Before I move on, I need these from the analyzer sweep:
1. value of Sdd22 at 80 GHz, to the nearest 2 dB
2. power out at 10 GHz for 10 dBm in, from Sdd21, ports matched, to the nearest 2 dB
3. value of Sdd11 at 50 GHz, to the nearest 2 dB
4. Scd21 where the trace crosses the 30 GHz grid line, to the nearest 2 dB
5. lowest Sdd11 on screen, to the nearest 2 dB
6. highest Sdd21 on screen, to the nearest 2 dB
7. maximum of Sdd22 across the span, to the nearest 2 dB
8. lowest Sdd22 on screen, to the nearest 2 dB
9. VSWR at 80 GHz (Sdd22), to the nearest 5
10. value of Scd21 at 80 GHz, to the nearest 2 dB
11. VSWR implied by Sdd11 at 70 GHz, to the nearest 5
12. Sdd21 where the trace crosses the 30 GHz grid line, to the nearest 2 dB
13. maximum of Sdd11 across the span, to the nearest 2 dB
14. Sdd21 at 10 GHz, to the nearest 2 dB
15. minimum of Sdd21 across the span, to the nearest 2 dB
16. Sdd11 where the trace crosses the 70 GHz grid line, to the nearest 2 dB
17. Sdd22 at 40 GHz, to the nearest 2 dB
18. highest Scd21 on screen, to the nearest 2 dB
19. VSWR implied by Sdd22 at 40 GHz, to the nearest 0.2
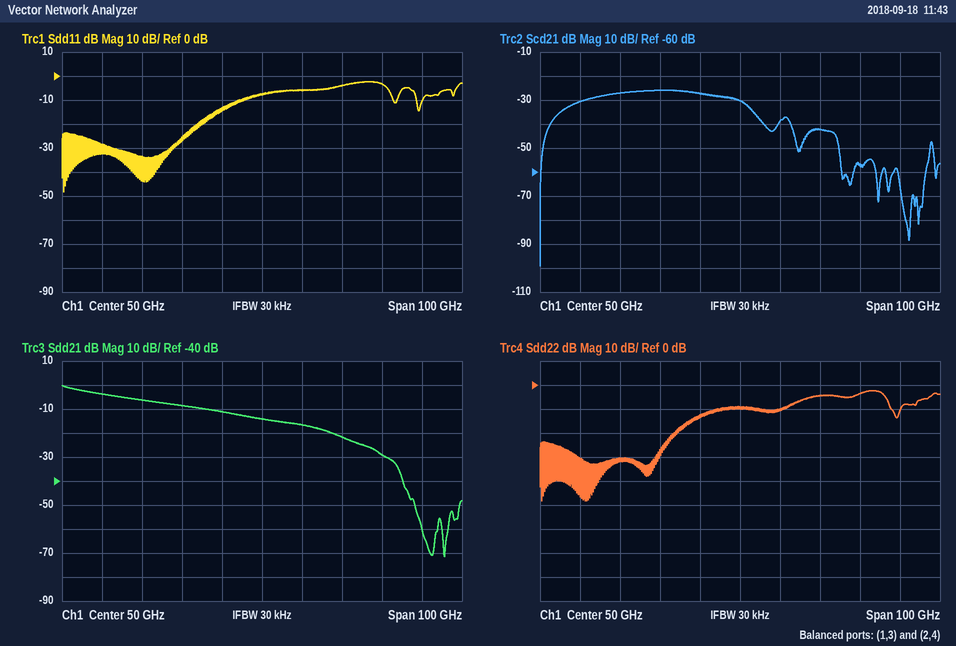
-4 dB
6 dBm
-8 dB
-26 dB
-48 dB
0 dB
-2 dB
-48 dB
5
-56 dB
5
-8 dB
-2 dB
-4 dB
-72 dB
-4 dB
-12 dB
-26 dB
1.6
